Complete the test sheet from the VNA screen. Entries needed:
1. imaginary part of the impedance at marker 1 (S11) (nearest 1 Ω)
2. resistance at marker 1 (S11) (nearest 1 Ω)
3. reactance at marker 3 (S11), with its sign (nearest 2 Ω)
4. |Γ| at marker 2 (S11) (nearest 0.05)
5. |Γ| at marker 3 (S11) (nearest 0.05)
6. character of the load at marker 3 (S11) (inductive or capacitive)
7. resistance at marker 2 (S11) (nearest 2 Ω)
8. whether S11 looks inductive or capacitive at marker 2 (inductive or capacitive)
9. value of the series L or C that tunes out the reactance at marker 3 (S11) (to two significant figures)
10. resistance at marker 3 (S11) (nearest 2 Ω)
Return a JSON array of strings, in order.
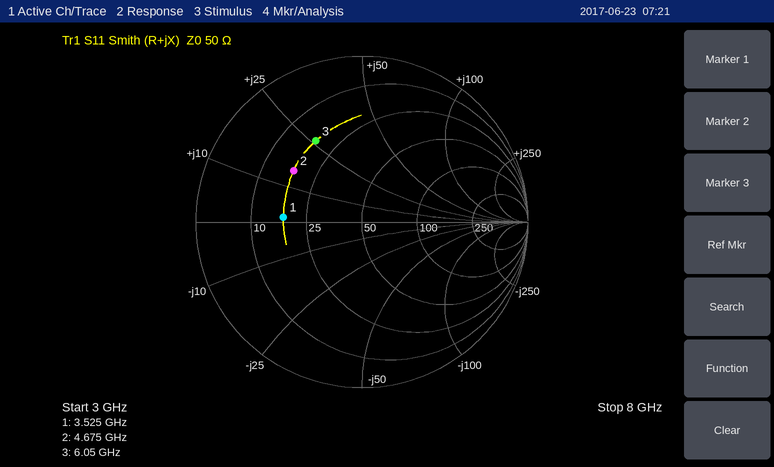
["+1 Ω", "18 Ω", "+26 Ω", "0.50", "0.55", "inductive", "18 Ω", "inductive", "1.0 pF", "18 Ω"]
